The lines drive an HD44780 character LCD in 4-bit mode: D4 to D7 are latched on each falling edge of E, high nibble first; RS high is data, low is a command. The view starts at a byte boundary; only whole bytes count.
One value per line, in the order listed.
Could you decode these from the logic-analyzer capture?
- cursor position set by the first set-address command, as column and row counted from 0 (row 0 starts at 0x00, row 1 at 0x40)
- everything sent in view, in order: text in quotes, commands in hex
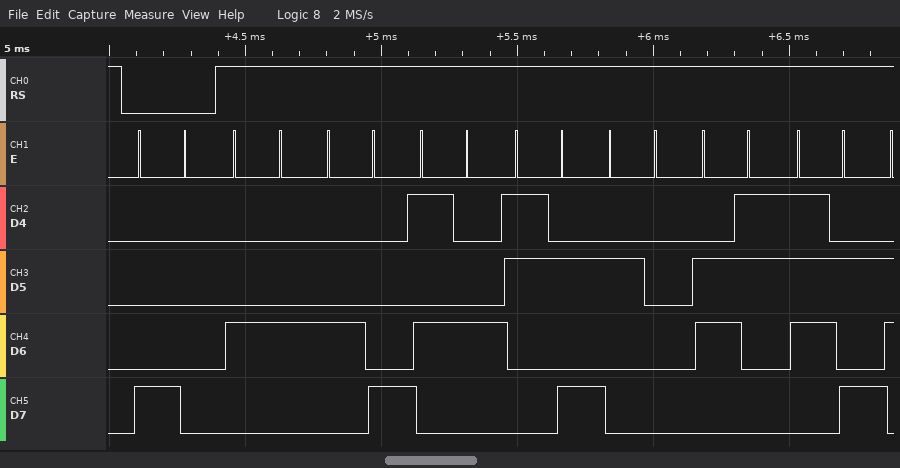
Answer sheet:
column 0, row 0
0x80 "DHT: cz"
